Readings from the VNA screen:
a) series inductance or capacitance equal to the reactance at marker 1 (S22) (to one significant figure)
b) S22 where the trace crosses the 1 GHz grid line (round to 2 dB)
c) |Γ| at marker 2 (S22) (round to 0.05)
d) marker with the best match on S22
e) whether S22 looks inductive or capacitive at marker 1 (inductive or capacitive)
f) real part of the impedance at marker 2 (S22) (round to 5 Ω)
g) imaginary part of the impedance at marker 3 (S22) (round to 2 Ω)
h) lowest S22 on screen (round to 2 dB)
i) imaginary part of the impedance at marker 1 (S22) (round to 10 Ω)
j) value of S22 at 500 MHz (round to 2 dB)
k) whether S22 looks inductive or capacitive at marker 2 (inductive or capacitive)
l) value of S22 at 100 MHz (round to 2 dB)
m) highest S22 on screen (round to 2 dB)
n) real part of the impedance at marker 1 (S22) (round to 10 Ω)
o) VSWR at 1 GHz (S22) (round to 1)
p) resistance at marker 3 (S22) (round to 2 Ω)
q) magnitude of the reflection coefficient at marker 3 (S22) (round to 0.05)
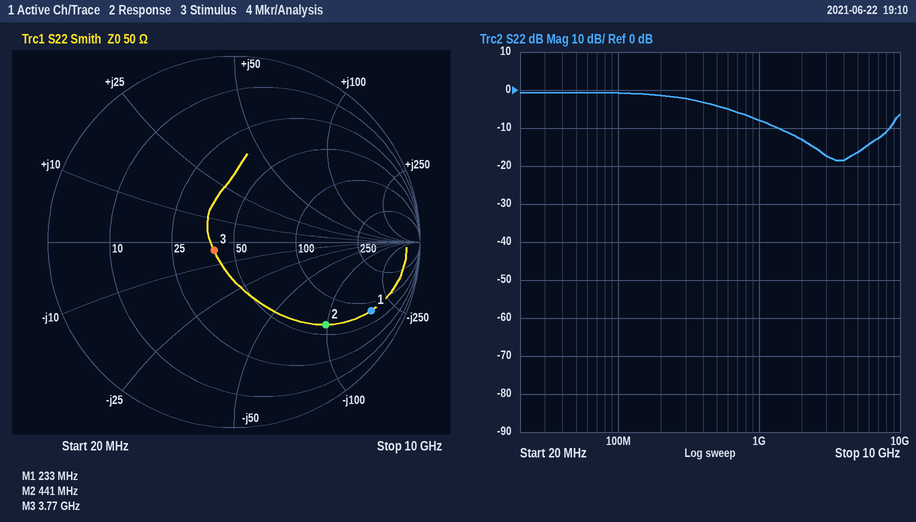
4 pF
-8 dB
0.65
marker 3
capacitive
60 Ω
-4 Ω
-18 dB
-180 Ω
-4 dB
capacitive
0 dB
0 dB
80 Ω
2
40 Ω
0.10
